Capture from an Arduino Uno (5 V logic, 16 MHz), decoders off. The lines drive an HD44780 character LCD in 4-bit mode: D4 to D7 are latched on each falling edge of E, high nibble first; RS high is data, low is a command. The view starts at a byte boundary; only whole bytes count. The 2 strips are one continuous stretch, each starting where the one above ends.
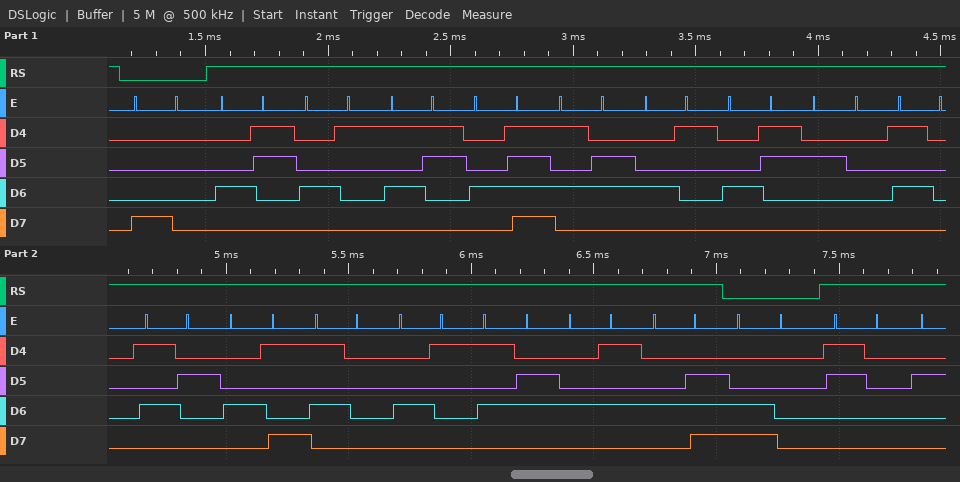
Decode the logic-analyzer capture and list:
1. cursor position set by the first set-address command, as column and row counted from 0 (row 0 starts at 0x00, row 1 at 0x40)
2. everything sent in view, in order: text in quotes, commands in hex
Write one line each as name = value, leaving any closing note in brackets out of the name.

cursor position set by the first set-address command, as column and row counted from 0 = column 0, row 0
everything sent in view, in order: text in quotes, commands in hex = 0x80 "CASOVAC PRIPAVEN" 0xC0 "0"
